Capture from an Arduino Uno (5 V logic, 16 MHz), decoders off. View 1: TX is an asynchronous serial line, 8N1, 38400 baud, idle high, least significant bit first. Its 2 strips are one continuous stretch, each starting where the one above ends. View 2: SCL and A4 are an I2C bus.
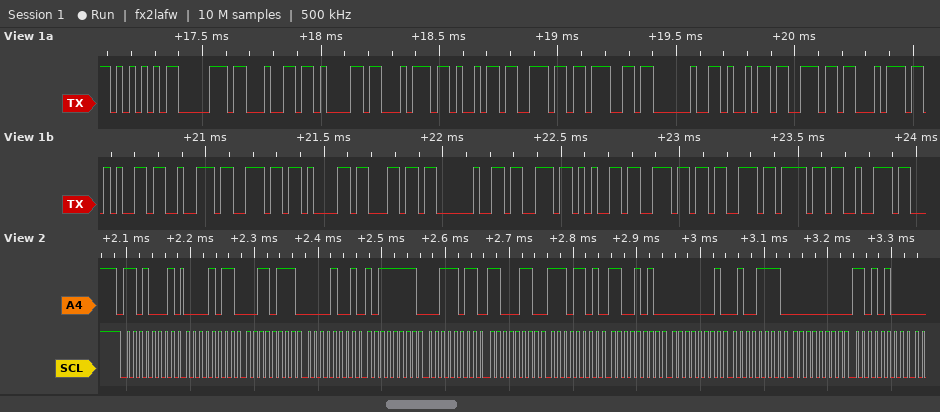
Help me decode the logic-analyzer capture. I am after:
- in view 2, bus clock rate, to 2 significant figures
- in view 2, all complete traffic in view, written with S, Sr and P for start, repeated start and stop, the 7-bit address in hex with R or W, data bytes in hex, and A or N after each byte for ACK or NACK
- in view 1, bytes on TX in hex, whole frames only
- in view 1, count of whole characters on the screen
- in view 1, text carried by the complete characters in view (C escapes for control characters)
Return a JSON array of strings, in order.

["100 kHz", "S 68R A 0B A 37 A 09 A BF A 3B A C6 A ED A CA A 01 A 4F A 00 A D4 A", "55 70 64 61 74 69 6E 67 20 69 6E 74 65 72 6E 61 6C 20 73 65 6E 73 6F 72", "24", "\"Updating internal sensor\""]
